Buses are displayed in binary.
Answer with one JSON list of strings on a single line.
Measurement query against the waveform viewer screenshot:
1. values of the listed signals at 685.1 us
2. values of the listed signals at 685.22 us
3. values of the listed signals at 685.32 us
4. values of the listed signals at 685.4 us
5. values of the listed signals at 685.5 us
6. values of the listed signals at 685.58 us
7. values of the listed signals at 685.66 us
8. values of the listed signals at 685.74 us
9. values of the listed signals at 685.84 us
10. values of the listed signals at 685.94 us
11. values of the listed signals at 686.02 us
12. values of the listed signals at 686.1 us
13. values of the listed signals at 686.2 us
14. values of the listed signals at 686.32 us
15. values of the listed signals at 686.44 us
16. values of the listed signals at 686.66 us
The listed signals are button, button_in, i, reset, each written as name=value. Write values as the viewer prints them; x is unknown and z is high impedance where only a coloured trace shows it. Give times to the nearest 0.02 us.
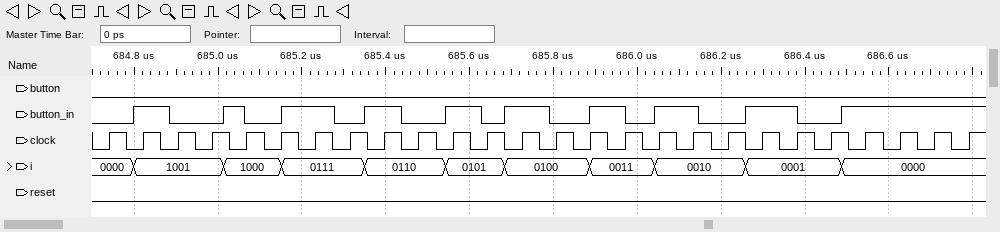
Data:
["button=0, button_in=0, i=1000, reset=0", "button=0, button_in=1, i=0111, reset=0", "button=0, button_in=0, i=0111, reset=0", "button=0, button_in=1, i=0110, reset=0", "button=0, button_in=0, i=0110, reset=0", "button=0, button_in=1, i=0101, reset=0", "button=0, button_in=0, i=0101, reset=0", "button=0, button_in=1, i=0100, reset=0", "button=0, button_in=0, i=0100, reset=0", "button=0, button_in=1, i=0011, reset=0", "button=0, button_in=0, i=0011, reset=0", "button=0, button_in=1, i=0010, reset=0", "button=0, button_in=0, i=0010, reset=0", "button=0, button_in=1, i=0001, reset=0", "button=0, button_in=0, i=0001, reset=0", "button=0, button_in=1, i=0000, reset=0"]
